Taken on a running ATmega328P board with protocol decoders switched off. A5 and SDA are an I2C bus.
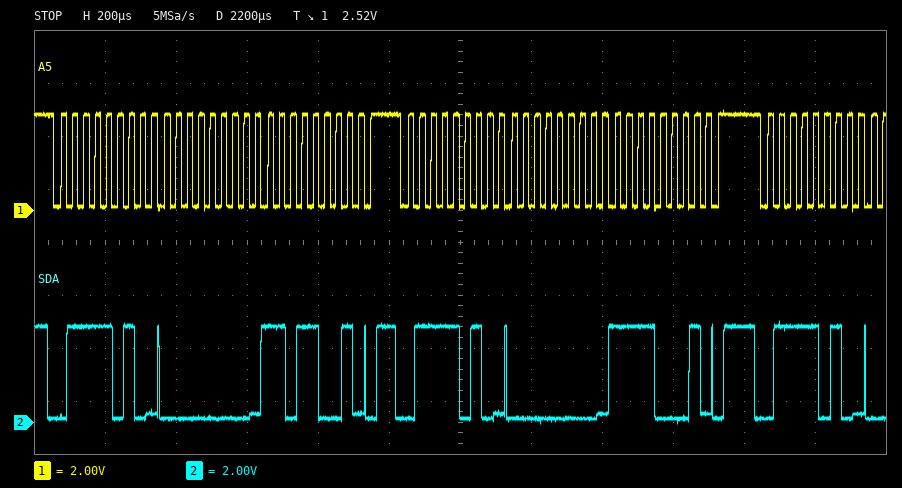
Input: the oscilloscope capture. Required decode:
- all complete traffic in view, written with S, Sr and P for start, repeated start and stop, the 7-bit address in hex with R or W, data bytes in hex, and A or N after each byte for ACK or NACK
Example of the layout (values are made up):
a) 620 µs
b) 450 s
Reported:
a) S 3DW A 00 A D9 A P S 3DW A 00 A F1 A P S 3DW A
